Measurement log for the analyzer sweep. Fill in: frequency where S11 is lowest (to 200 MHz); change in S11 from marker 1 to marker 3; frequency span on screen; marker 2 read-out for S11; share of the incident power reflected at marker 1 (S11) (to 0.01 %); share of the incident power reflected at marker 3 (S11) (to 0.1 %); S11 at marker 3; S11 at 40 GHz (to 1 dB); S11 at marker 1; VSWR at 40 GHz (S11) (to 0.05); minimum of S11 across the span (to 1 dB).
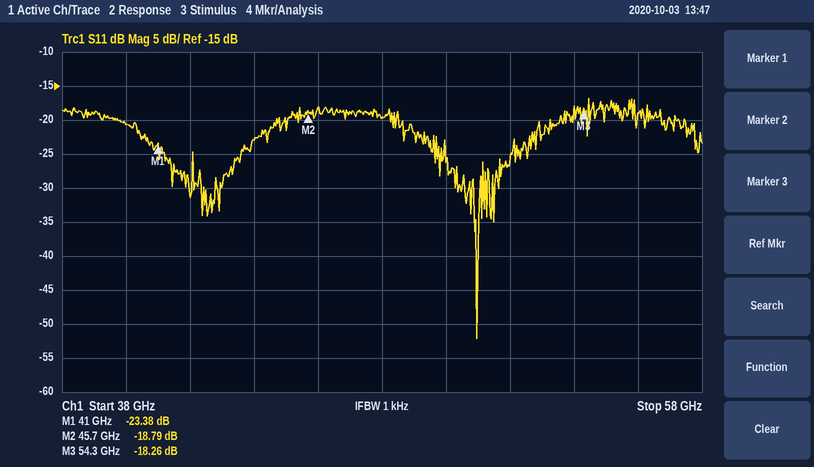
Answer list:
51.0 GHz
5.12 dB
20 GHz
-18.79 dB
0.46 %
1.5 %
-18.26 dB
-21 dB
-23.38 dB
1.20
-52 dB
